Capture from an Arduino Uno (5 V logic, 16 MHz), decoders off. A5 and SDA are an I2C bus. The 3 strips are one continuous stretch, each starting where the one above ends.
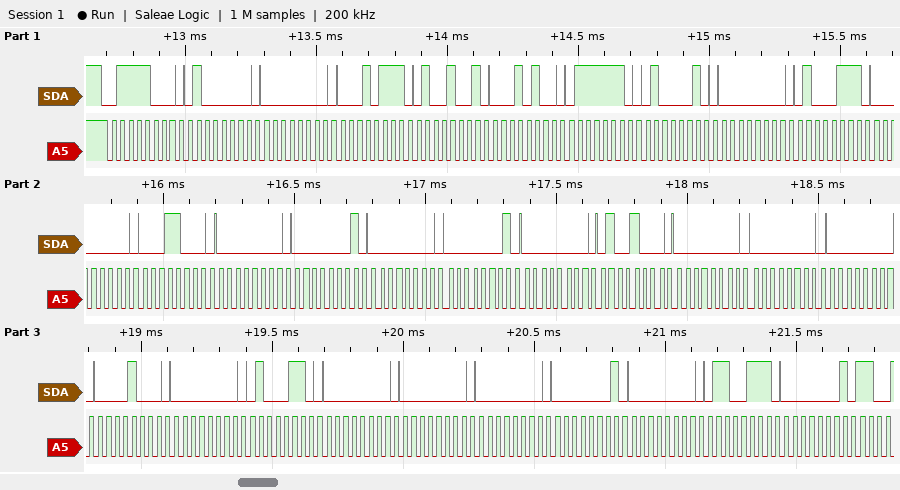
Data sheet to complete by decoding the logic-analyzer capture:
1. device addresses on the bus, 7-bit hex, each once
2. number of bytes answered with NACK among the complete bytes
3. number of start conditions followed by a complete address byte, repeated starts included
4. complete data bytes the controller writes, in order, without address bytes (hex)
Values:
0x3C
0
1
40 00 17 49 14 7E 42 00 47 00 18 00 01 00 01 00 48 00 00 00 08 00 46 00 00 00 01 00 67 01
